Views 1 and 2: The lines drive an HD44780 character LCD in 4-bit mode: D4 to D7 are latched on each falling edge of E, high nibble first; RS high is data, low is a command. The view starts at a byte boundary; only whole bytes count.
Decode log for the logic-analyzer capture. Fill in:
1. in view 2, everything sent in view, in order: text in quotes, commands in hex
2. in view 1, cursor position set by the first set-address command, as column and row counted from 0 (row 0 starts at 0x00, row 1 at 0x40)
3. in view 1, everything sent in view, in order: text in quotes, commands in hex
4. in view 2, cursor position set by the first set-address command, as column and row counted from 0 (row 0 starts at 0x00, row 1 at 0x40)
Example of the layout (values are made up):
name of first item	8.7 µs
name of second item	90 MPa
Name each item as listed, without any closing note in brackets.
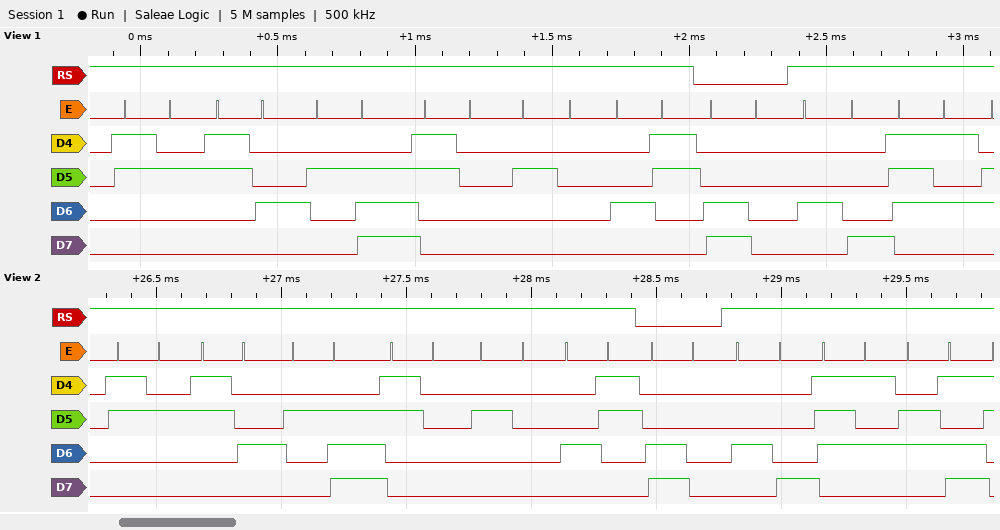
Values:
in view 2, everything sent in view, in order: text in quotes, commands in hex	"24.0 C" 0xC0 "Hum"
in view 1, cursor position set by the first set-address command, as column and row counted from 0	column 0, row 1
in view 1, everything sent in view, in order: text in quotes, commands in hex	"24.0 C" 0xC0 "Hu"
in view 2, cursor position set by the first set-address command, as column and row counted from 0	column 0, row 1
